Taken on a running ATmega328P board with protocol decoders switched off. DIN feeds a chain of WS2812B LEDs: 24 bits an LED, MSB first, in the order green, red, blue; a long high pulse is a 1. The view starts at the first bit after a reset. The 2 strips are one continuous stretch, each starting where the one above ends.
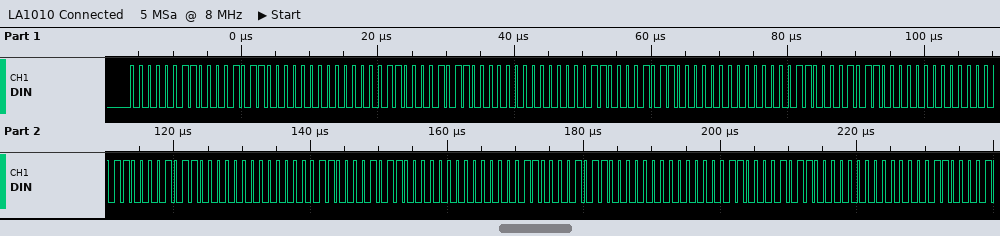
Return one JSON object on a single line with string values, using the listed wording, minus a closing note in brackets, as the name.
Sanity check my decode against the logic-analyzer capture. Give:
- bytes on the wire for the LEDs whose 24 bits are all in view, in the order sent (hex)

{"bytes on the wire for the LEDs whose 24 bits are all in view, in the order sent": "03 0B 00 03 0B 00 03 0B 00 03 0B 00 03 0B 00 03 0B 00 03 0B 00 03 0B 00"}
